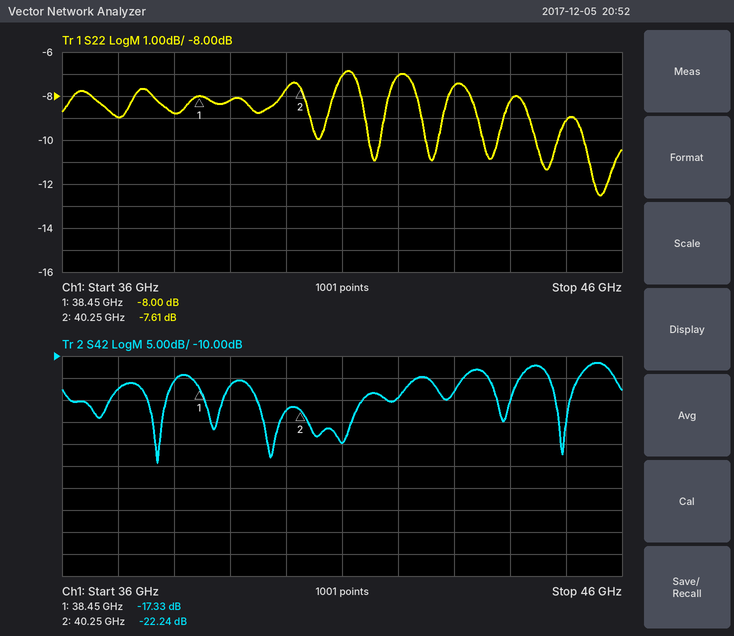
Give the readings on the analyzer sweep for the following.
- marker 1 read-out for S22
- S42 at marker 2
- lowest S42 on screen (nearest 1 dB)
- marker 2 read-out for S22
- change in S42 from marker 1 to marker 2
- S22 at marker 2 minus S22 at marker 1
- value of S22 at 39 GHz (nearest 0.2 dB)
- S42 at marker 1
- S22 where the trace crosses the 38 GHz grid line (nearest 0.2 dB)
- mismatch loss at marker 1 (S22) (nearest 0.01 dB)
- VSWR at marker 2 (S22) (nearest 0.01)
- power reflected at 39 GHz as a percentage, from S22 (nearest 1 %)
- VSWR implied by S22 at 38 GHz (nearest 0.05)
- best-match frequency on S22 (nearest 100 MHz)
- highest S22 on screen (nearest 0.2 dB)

-8.00 dB
-22.24 dB
-34 dB
-7.61 dB
-4.91 dB
0.39 dB
-8.2 dB
-17.33 dB
-8.8 dB
0.75 dB
2.43
15 %
2.15
45.6 GHz
-6.8 dB
